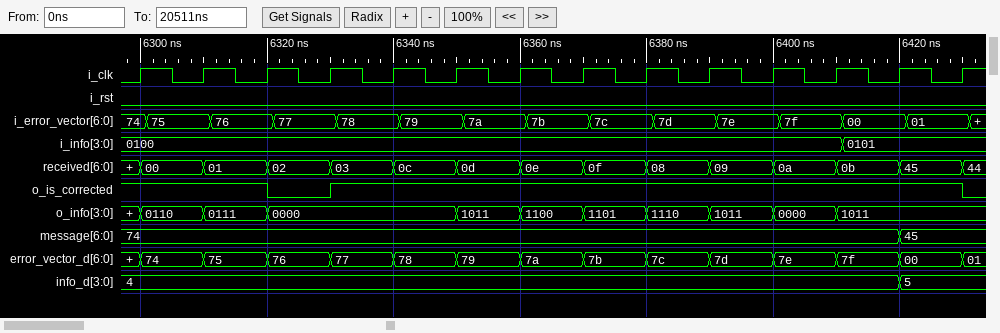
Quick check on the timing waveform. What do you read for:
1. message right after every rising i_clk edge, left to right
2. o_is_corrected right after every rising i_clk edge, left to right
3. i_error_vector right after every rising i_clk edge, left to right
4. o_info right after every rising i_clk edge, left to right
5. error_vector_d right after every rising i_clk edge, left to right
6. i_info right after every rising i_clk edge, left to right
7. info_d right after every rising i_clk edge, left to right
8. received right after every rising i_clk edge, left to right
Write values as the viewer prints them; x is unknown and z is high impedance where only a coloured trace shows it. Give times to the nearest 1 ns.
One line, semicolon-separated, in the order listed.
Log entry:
74, 74, 74, 74, 74, 74, 74, 74, 74, 74, 74, 74, 45, 45; 1 1 0 1 1 1 1 1 1 1 1 1 1 0; 74, 75, 76, 77, 78, 79, 7a, 7b, 7c, 7d, 7e, 7f, 00, 01; 0110, 0111, 0000, 0000, 0000, 1011, 1100, 1101, 1110, 1011, 0000, 1011, 1011, 1011; 74, 75, 76, 77, 78, 79, 7a, 7b, 7c, 7d, 7e, 7f, 00, 01; 0100, 0100, 0100, 0100, 0100, 0100, 0100, 0100, 0100, 0100, 0100, 0100, 0101, 0101; 4, 4, 4, 4, 4, 4, 4, 4, 4, 4, 4, 4, 5, 5; 00, 01, 02, 03, 0c, 0d, 0e, 0f, 08, 09, 0a, 0b, 45, 44
